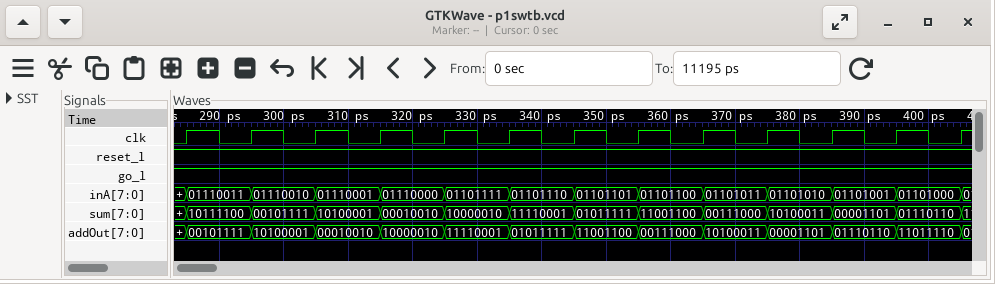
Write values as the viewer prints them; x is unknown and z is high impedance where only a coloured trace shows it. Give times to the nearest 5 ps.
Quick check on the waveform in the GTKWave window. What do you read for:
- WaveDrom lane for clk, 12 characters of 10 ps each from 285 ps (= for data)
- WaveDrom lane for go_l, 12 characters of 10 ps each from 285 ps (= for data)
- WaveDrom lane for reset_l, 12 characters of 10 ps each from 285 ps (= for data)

{name: 'clk', wave: 'p...........'}
{name: 'go_l', wave: '1...........'}
{name: 'reset_l', wave: '1...........'}
